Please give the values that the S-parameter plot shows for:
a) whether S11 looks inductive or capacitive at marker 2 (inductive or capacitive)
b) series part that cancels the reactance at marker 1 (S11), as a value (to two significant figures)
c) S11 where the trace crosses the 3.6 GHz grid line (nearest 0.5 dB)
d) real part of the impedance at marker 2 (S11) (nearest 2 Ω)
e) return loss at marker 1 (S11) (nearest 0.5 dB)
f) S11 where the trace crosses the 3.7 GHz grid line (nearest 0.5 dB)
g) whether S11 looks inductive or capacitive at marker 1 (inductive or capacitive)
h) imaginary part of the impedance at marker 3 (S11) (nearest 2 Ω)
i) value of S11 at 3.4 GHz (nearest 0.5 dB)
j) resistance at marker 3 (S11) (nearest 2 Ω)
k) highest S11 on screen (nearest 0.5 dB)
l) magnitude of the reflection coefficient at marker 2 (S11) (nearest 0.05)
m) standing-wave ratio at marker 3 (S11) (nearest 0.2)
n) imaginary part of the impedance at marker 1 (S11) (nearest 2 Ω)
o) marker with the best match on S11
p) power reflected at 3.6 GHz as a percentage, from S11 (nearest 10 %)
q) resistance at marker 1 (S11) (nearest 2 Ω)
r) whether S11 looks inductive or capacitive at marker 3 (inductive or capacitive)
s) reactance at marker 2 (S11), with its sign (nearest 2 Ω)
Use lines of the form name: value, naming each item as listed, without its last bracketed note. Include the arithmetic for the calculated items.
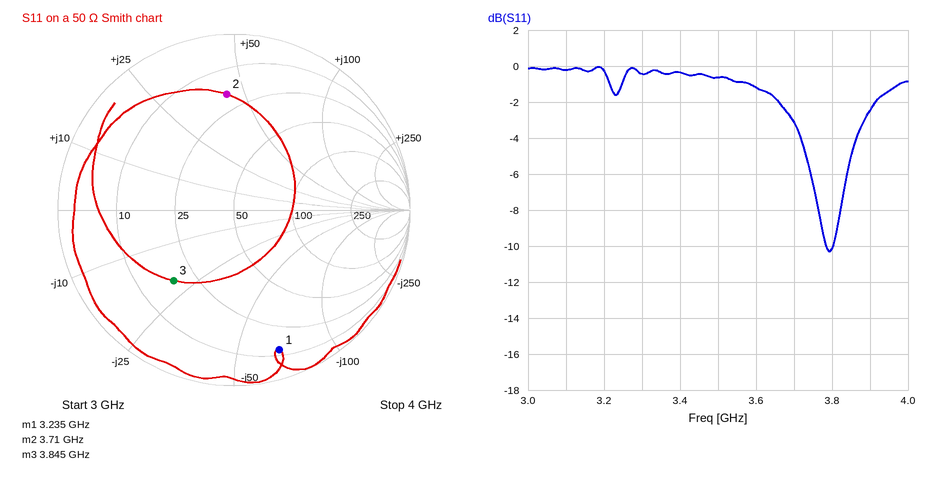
whether S11 looks inductive or capacitive at marker 2: inductive
series part that cancels the reactance at marker 1 (S11), as a value: L = 68 Ω/(2π × 3.235 GHz) ≈ 3.3 nH
S11 where the trace crosses the 3.6 GHz grid line: -1.0 dB
real part of the impedance at marker 2 (S11): 18 Ω
return loss at marker 1 (S11): 1.5 dB
S11 where the trace crosses the 3.7 GHz grid line: -3.0 dB
whether S11 looks inductive or capacitive at marker 1: capacitive
imaginary part of the impedance at marker 3 (S11): -20 Ω
value of S11 at 3.4 GHz: -0.5 dB
resistance at marker 3 (S11): 18 Ω
highest S11 on screen: 0.0 dB
magnitude of the reflection coefficient at marker 2 (S11): 0.65
standing-wave ratio at marker 3 (S11): 3.2
imaginary part of the impedance at marker 1 (S11): -68 Ω
marker with the best match on S11: marker 3
power reflected at 3.6 GHz as a percentage, from S11: 10^(-1/10) ≈ 79.4 %, so 80 % to the nearest 10 %
resistance at marker 1 (S11): 12 Ω
whether S11 looks inductive or capacitive at marker 3: capacitive
reactance at marker 2 (S11), with its sign: +44 Ω
